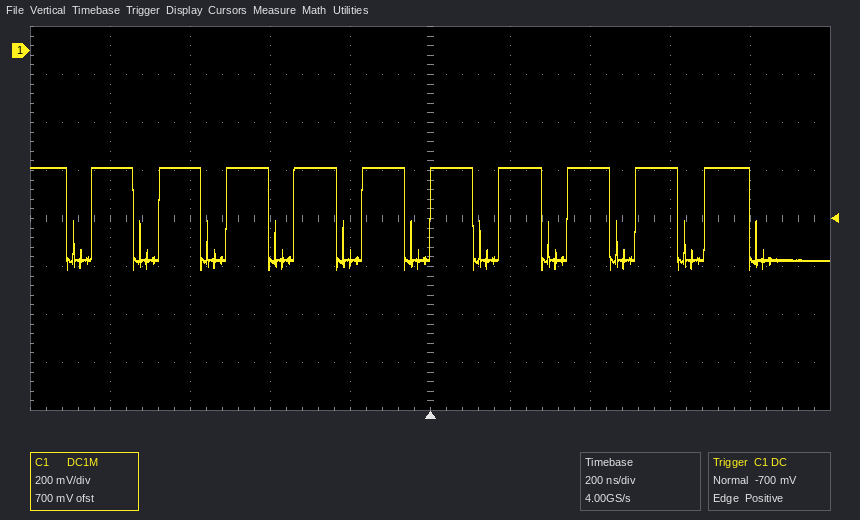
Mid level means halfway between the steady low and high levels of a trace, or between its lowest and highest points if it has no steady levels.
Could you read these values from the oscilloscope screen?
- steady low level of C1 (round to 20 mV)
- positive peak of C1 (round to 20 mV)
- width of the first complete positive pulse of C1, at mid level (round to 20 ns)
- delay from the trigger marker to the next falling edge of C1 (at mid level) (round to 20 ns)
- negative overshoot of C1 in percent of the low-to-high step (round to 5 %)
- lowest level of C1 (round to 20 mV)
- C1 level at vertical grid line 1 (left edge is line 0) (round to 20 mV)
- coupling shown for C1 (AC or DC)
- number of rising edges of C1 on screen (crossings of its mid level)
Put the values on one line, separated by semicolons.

-880 mV; -480 mV; 100 ns; 100 ns; 10 %; -920 mV; -480 mV; DC; 10
